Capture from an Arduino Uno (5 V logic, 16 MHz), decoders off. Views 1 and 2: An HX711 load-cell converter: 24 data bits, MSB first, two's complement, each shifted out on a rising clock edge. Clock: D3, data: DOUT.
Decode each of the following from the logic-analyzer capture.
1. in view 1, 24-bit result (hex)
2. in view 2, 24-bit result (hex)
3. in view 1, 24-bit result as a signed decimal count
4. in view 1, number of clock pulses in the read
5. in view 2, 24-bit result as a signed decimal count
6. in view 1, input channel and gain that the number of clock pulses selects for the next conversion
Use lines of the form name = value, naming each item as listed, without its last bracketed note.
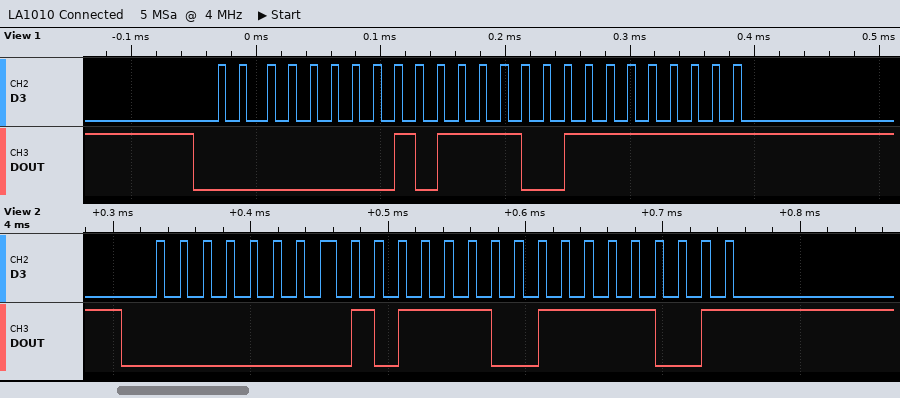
in view 1, 24-bit result = 0x00BCFF
in view 2, 24-bit result = 0x00BCF9
in view 1, 24-bit result as a signed decimal count = 48383
in view 1, number of clock pulses in the read = 25
in view 2, 24-bit result as a signed decimal count = 48377
in view 1, input channel and gain that the number of clock pulses selects for the next conversion = channel A, gain 128
